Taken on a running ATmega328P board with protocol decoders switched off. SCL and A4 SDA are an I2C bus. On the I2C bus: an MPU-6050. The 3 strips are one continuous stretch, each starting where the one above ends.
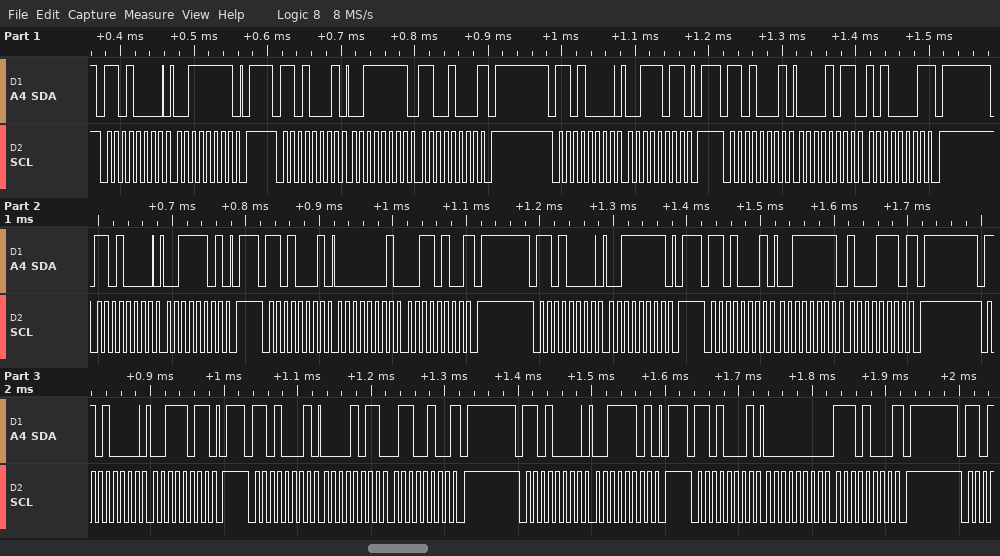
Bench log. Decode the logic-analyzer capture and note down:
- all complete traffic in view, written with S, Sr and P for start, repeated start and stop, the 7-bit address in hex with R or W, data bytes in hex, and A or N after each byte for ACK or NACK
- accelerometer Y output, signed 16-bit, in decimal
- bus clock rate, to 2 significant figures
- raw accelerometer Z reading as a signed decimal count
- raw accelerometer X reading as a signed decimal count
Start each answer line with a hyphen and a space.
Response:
- S 68W A 3F A P S 68R A 3F A C8 N P S 68W A 3B A P S 68R A 0B A A1 N P S 68W A 3D A P S 68R A 01 A 34 N P S 68W A 3F A P S 68R A 3F A 8E N P S 68W A 3B A P S 68R A 0B A 64 N P S 68W A 3D A P S 68R A 00 A E8 N P
- 308
- 100 kHz
- 16328
- 2977
